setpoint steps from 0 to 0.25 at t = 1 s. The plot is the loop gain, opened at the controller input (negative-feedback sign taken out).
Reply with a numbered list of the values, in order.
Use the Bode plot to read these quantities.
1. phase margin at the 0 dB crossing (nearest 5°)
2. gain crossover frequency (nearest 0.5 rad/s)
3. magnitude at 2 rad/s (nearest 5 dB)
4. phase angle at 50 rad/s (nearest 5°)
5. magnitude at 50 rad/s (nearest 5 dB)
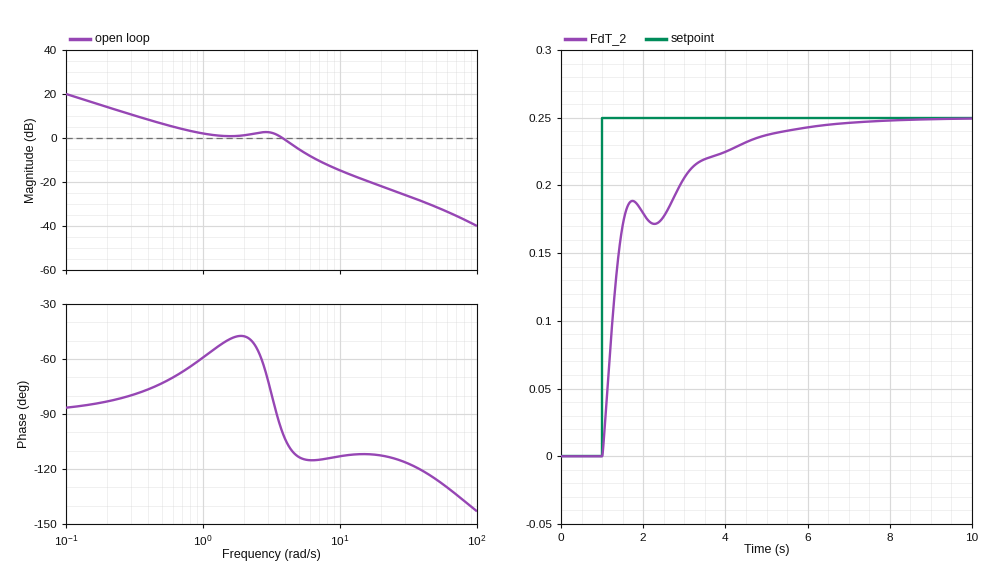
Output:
1. 80°
2. 4.0 rad/s
3. 0 dB
4. -125°
5. -30 dB
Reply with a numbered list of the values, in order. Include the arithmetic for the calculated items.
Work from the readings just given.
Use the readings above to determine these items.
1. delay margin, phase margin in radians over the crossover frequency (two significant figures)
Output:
1. 80 × π / 180 / 4 = 0.35 s
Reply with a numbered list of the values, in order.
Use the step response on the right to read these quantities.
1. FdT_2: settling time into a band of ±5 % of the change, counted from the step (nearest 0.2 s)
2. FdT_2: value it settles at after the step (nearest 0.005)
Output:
1. 4.0 s
2. 0.250
